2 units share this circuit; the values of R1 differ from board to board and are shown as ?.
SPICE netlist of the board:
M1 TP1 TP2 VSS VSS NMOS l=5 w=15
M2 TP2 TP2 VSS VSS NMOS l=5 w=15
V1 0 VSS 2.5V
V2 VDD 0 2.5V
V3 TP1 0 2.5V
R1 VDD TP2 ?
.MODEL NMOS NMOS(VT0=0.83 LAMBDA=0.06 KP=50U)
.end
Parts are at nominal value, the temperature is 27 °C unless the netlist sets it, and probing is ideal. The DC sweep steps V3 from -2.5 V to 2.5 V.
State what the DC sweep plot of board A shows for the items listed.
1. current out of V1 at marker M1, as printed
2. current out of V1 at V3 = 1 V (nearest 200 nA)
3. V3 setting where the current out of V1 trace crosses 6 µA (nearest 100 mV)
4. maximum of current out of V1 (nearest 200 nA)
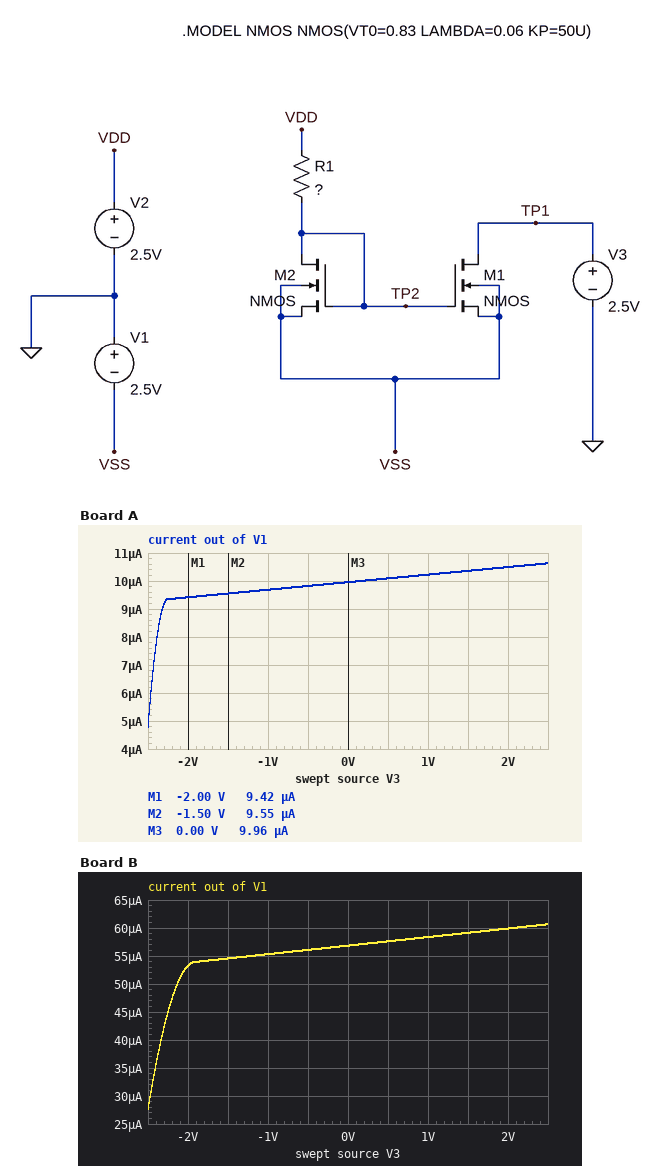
9.42 µA
10.2 µA
-2.5 V
10.6 µA
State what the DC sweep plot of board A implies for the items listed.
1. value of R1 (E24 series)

820 kΩ
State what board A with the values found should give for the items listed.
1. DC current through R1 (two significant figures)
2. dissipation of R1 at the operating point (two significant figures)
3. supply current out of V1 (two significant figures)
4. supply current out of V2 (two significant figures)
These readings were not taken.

4.8 µA
19 µW
11 µA
4.8 µA
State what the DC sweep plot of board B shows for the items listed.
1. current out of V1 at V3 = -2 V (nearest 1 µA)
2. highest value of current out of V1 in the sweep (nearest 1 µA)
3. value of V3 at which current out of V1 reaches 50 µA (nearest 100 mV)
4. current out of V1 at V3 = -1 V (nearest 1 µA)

53 µA
61 µA
-2.1 V
55 µA
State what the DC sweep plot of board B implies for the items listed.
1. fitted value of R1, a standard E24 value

130 kΩ
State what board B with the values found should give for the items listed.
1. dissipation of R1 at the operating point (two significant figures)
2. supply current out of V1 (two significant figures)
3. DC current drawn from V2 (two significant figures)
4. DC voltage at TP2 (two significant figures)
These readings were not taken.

99 µW
61 µA
28 µA
-1.1 V
